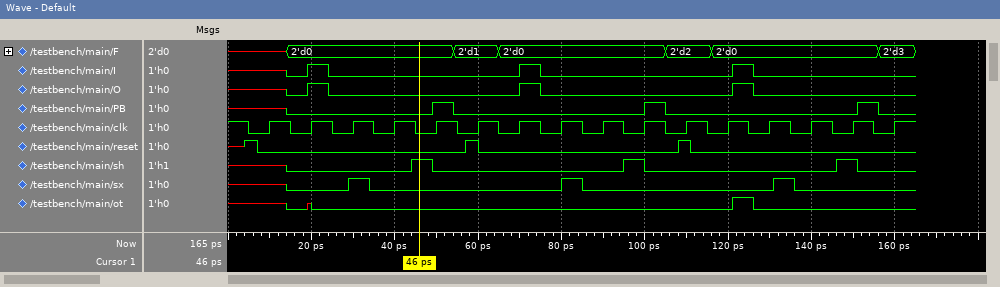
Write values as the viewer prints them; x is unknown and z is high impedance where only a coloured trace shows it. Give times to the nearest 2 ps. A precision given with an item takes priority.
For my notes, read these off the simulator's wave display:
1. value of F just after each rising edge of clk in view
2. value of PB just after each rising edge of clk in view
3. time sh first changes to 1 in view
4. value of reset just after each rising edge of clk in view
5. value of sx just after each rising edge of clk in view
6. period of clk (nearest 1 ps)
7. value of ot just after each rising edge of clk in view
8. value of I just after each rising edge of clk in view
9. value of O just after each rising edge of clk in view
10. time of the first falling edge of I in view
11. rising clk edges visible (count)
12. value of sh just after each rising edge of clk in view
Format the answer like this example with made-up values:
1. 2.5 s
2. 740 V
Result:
1. x, 2'd0, 2'd0, 2'd0, 2'd0, 2'd1, 2'd0, 2'd0, 2'd0, 2'd0, 2'd2, 2'd0, 2'd0, 2'd0, 2'd0, 2'd3
2. x 0 0 0 1 0 0 0 0 1 0 0 0 0 0 0
3. 44 ps
4. 0 0 0 0 0 0 0 0 0 0 1 0 0 0 0 0
5. x 0 1 0 0 0 0 1 0 0 0 0 0 0 0 0
6. 10 ps
7. x 0 0 0 0 0 0 0 0 0 0 0 0 0 0 0
8. x 1 0 0 0 0 1 0 0 0 0 0 0 0 0 0
9. x 1 0 0 0 0 1 0 0 0 0 0 0 0 0 0
10. 24 ps
11. 16
12. x 0 0 0 0 0 0 0 0 0 0 0 0 0 1 0
